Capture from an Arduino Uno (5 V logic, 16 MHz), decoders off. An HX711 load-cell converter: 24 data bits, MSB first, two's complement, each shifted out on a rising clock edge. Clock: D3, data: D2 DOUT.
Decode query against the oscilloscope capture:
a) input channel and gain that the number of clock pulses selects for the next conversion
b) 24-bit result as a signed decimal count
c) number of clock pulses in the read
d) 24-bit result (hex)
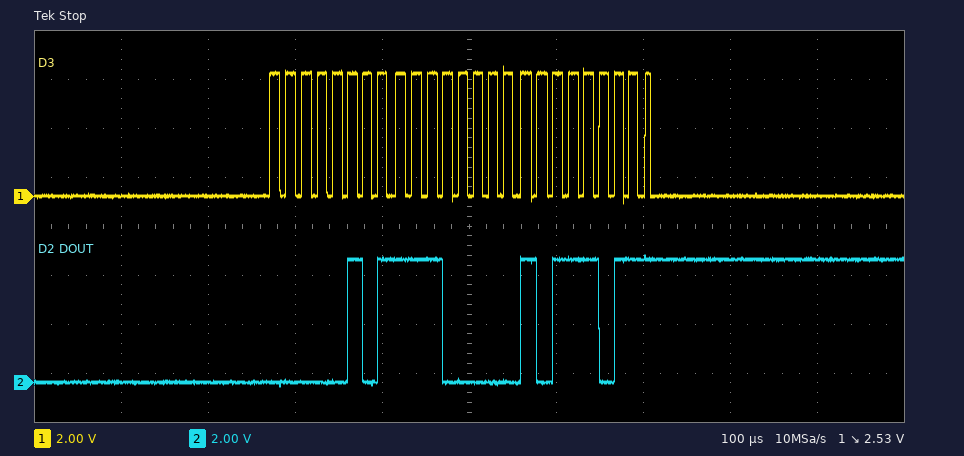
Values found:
channel A, gain 128
385211
25
0x05E0BB
